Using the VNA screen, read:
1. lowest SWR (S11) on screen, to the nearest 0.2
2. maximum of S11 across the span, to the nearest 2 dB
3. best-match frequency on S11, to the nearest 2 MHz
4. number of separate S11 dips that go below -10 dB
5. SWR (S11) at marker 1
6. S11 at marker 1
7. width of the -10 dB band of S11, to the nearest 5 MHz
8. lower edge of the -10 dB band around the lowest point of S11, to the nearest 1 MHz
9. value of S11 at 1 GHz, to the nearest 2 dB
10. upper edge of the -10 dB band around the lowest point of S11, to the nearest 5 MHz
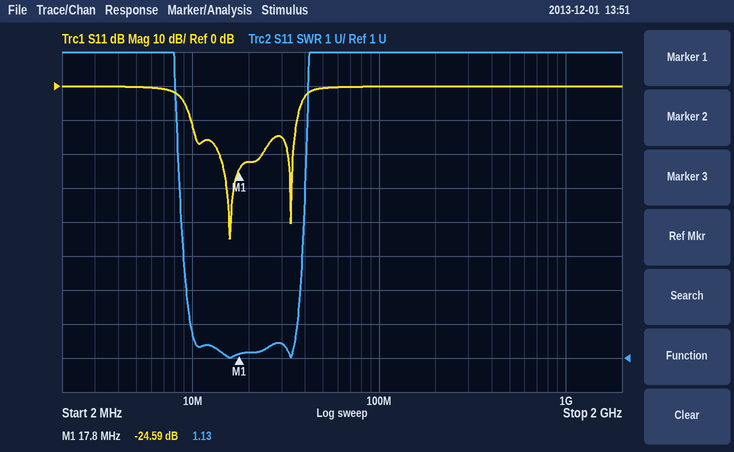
1.0
0 dB
16 MHz
2
1.13
-24.59 dB
25 MHz
10 MHz
0 dB
35 MHz
